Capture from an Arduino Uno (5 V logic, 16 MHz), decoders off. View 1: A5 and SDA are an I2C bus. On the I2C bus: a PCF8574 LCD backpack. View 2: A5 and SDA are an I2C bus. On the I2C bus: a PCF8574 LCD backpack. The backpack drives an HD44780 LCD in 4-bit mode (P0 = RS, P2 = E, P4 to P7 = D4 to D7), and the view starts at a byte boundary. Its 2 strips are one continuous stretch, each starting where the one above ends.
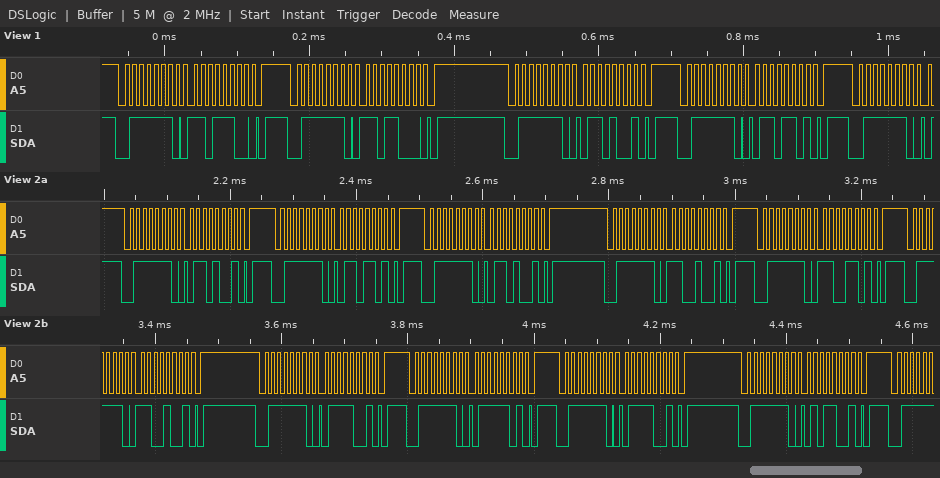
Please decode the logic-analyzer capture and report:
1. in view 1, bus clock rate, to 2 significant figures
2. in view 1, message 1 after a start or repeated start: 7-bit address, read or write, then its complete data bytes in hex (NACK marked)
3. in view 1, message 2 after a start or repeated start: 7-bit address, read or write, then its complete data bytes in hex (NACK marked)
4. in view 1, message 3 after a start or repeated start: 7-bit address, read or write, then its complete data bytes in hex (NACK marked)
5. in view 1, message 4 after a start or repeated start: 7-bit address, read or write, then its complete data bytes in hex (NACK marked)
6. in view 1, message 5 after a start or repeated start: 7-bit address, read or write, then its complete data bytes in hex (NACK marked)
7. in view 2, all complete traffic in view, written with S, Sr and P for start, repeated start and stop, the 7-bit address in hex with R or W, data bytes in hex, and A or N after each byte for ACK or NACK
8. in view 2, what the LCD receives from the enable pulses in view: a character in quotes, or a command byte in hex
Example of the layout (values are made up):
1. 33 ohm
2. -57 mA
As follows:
1. 100 kHz
2. 0x3F write: DC
3. 0x3F write: D8
4. 0x3F write: 69
5. 0x3F write: 6D
6. 0x3F write
7. S 3FW A 69 A P S 3FW A 6D A P S 3FW A 69 A P S 3FW A C9 A P S 3FW A CD A P S 3FW A C9 A P S 3FW A 79 A P S 3FW A 7D A P S 3FW A 79 A P S 3FW A 59 A P
8. 'l'
